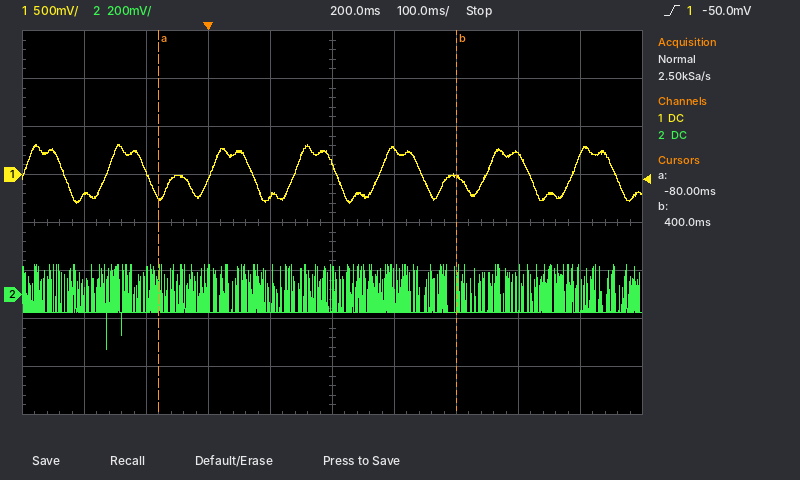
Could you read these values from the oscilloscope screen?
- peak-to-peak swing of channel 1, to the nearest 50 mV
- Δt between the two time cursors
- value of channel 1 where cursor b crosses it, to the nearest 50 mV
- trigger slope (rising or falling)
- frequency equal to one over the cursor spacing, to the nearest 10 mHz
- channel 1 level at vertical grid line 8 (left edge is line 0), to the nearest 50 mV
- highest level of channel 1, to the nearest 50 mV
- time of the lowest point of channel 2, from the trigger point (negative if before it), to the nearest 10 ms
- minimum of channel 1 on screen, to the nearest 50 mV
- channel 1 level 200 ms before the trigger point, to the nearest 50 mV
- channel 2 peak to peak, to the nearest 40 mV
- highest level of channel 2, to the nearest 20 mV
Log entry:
600 mV
480 ms
0 mV
rising
2.08 Hz
200 mV
300 mV
-160 ms
-300 mV
-200 mV
360 mV
120 mV
